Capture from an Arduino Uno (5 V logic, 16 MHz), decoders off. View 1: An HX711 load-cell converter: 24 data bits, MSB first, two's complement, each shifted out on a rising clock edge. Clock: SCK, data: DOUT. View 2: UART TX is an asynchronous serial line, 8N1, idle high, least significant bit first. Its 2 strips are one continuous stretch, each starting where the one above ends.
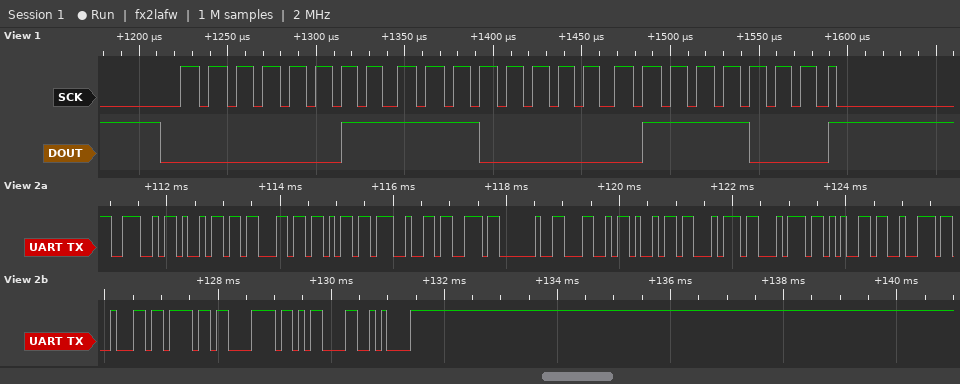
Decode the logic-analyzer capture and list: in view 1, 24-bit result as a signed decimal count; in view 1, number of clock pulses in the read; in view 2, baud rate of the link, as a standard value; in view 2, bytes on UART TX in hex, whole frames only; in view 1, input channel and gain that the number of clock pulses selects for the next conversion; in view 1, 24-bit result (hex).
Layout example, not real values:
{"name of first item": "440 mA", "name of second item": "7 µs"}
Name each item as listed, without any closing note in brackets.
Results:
{"in view 1, 24-bit result as a signed decimal count": "254072", "in view 1, number of clock pulses in the read": "25", "in view 2, baud rate of the link, as a standard value": "9600 baud", "in view 2, bytes on UART TX in hex, whole frames only": "0x4E 0x69 0x63 0x6B 0x27 0x73 0x20 0x4C 0x69 0x74 0x74 0x65 0x72 0x62 0x6F 0x78 0x0D 0x0A", "in view 1, input channel and gain that the number of clock pulses selects for the next conversion": "channel A, gain 128", "in view 1, 24-bit result": "0x03E078"}
